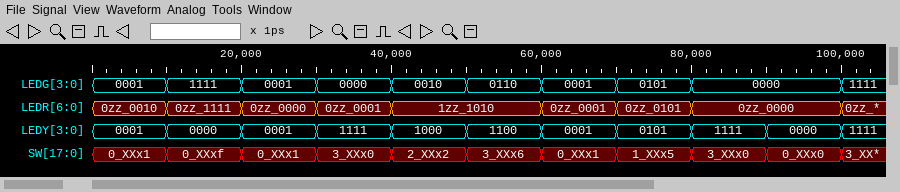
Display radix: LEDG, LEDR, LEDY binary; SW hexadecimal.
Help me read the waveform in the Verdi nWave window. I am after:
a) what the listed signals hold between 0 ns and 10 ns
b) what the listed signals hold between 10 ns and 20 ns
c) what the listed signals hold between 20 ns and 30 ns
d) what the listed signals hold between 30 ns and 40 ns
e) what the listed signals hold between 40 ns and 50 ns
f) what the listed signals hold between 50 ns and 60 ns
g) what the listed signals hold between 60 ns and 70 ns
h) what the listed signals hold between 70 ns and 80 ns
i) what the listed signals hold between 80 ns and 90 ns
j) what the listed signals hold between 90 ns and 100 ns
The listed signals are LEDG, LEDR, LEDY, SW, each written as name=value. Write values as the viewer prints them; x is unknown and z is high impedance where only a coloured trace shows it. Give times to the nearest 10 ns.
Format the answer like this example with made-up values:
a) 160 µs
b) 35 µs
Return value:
a) LEDG=0001, LEDR=0zz_0010, LEDY=0001, SW=0_XXx1
b) LEDG=1111, LEDR=0zz_1111, LEDY=0000, SW=0_XXxf
c) LEDG=0001, LEDR=0zz_0000, LEDY=0001, SW=0_XXx1
d) LEDG=0000, LEDR=0zz_0001, LEDY=1111, SW=3_XXx0
e) LEDG=0010, LEDR=1zz_1010, LEDY=1000, SW=2_XXx2
f) LEDG=0110, LEDR=1zz_1010, LEDY=1100, SW=3_XXx6
g) LEDG=0001, LEDR=0zz_0001, LEDY=0001, SW=0_XXx1
h) LEDG=0101, LEDR=0zz_0101, LEDY=0101, SW=1_XXx5
i) LEDG=0000, LEDR=0zz_0000, LEDY=1111, SW=3_XXx0
j) LEDG=0000, LEDR=0zz_0000, LEDY=0000, SW=0_XXx0
